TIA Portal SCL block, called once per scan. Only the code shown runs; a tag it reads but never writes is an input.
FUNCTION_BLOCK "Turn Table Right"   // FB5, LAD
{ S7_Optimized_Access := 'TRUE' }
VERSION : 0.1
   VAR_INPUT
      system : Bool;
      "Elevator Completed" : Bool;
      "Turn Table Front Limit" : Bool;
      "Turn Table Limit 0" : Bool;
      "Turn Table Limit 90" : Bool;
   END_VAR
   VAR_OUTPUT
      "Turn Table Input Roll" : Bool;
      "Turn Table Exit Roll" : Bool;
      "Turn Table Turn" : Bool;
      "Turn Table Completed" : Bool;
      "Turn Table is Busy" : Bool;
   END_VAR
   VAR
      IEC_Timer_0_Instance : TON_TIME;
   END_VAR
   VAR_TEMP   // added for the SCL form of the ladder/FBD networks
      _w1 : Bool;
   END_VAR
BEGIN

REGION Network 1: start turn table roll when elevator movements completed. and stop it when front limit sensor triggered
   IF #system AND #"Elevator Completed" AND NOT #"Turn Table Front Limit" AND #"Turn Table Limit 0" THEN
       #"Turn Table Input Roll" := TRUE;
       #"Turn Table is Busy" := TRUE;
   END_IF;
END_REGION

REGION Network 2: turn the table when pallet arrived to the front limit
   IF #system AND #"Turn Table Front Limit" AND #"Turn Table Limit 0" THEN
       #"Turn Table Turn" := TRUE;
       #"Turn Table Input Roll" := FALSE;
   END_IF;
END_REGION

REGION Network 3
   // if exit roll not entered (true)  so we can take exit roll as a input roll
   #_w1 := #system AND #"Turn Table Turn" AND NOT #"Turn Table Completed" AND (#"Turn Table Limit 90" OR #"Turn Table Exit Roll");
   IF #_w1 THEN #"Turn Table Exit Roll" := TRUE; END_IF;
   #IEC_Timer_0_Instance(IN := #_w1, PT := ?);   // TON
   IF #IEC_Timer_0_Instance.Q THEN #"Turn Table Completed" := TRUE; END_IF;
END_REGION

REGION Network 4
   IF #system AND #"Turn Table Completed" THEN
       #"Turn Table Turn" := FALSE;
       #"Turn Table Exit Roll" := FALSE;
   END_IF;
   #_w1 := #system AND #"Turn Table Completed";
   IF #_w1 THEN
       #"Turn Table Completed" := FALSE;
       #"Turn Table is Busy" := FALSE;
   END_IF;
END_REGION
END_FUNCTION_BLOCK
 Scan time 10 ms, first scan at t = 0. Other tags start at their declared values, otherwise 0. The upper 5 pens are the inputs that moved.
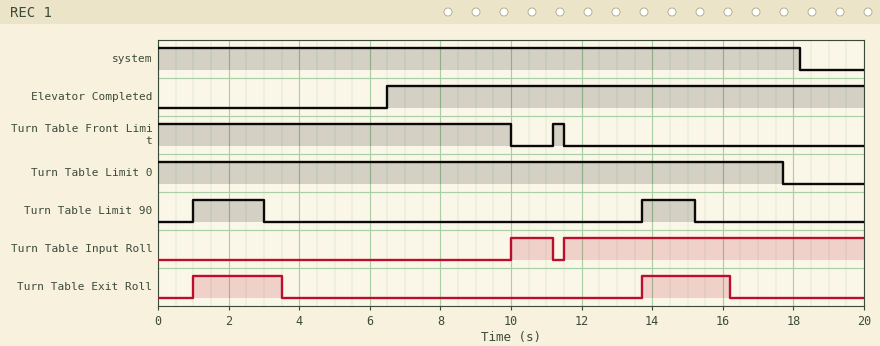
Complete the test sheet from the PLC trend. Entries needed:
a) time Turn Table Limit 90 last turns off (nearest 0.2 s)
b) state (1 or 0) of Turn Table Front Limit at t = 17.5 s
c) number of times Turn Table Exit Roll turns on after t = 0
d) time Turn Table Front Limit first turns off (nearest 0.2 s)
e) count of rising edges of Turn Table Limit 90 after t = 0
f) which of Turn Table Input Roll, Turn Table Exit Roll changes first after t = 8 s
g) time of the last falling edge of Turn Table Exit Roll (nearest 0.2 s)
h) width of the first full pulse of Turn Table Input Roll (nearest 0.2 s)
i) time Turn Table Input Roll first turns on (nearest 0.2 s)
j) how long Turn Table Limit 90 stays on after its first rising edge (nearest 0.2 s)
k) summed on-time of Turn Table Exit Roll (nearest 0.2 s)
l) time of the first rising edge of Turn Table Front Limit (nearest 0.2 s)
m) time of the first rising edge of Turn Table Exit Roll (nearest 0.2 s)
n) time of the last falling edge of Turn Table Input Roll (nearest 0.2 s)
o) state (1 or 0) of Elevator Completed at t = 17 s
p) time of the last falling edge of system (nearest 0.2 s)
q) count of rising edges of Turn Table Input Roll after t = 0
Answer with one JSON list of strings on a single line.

["15.2 s", "0", "2", "10.0 s", "2", "Turn Table Input Roll", "16.2 s", "1.2 s", "10.0 s", "2.0 s", "5.0 s", "11.2 s", "1.0 s", "11.2 s", "1", "18.2 s", "2"]
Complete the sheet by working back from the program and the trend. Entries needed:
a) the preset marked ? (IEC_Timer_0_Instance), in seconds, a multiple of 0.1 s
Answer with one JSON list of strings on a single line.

["2.5 s"]
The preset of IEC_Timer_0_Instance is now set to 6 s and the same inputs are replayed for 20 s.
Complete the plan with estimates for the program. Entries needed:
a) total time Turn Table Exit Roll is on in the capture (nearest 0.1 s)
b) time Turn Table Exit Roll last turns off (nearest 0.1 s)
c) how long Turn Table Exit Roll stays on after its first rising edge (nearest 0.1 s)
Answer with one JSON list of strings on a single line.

["12.3 s", "7.0 s", "6.0 s"]
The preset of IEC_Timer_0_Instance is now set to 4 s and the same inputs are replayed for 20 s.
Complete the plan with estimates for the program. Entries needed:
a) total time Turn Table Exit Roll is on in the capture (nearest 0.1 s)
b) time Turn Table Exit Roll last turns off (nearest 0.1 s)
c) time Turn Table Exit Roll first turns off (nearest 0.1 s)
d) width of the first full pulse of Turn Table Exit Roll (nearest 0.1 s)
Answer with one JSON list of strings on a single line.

["8.0 s", "17.7 s", "5.0 s", "4.0 s"]
